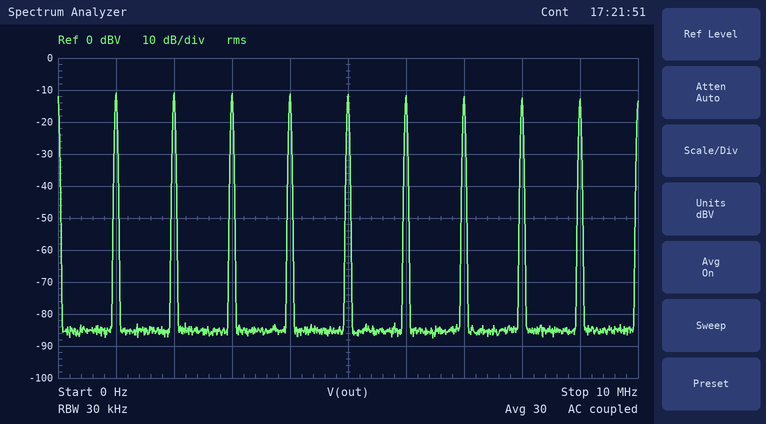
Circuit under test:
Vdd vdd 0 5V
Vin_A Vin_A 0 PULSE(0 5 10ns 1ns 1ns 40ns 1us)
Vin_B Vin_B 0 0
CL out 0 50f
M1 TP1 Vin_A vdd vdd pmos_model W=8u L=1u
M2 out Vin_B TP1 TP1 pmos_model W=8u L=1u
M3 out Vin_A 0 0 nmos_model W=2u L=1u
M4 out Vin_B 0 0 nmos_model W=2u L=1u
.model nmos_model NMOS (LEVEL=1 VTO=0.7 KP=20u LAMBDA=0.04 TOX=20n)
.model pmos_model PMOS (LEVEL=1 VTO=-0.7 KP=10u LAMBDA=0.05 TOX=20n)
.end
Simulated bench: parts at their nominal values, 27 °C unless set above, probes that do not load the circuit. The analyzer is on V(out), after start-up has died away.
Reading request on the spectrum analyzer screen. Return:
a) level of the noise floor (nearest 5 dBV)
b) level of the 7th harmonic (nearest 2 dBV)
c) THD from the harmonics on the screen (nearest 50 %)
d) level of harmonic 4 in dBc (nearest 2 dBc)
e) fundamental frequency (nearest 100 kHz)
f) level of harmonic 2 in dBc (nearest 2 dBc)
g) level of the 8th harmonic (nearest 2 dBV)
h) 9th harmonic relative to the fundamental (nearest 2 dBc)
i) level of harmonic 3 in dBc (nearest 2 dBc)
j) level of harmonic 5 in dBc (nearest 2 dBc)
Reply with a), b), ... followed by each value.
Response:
a) -85 dBV
b) -12 dBV
c) 250 %
d) 0 dBc
e) 1.0 MHz
f) 0 dBc
g) -12 dBV
h) -2 dBc
i) 0 dBc
j) 0 dBc
